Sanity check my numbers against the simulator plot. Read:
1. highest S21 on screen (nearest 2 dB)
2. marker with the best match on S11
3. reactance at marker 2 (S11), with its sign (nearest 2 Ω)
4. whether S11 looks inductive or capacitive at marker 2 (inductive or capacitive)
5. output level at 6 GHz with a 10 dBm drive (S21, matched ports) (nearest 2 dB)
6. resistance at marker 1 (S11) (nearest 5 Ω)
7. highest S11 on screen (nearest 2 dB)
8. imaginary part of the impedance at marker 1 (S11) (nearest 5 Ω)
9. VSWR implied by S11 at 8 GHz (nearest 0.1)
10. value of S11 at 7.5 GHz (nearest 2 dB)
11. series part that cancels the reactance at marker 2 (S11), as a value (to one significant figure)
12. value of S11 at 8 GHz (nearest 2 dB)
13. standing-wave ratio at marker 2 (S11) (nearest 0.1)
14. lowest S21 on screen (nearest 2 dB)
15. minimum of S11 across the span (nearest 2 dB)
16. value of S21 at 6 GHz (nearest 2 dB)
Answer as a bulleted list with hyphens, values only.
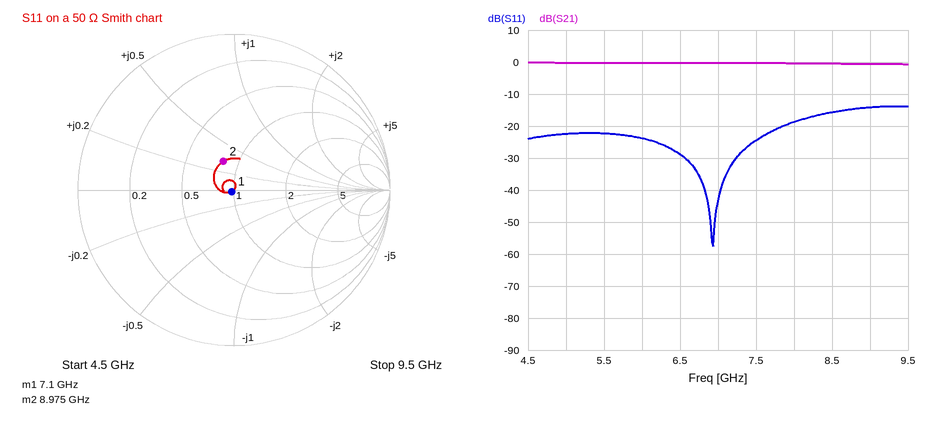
- 0 dB
- marker 1
- +16 Ω
- inductive
- 10 dBm
- 50 Ω
- -14 dB
- 0 Ω
- 1.3
- -24 dB
- 1 pF
- -18 dB
- 1.5
- 0 dB
- -58 dB
- 0 dB
